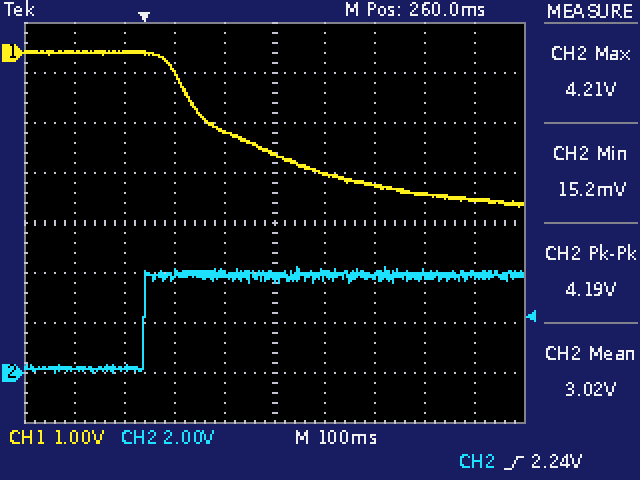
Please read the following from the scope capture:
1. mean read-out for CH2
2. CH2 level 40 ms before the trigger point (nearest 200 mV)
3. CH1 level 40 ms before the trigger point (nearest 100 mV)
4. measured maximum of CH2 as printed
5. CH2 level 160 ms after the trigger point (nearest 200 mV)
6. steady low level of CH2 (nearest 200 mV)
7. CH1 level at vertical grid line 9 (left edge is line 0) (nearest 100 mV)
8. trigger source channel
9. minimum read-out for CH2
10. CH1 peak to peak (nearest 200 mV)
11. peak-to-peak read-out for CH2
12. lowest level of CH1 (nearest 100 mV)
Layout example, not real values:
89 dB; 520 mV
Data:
3.02 V; 200 mV; 0.0 V; 4.21 V; 4.0 V; 200 mV; -2.9 V; CH2; 15.2 mV; 3.2 V; 4.19 V; -3.1 V
